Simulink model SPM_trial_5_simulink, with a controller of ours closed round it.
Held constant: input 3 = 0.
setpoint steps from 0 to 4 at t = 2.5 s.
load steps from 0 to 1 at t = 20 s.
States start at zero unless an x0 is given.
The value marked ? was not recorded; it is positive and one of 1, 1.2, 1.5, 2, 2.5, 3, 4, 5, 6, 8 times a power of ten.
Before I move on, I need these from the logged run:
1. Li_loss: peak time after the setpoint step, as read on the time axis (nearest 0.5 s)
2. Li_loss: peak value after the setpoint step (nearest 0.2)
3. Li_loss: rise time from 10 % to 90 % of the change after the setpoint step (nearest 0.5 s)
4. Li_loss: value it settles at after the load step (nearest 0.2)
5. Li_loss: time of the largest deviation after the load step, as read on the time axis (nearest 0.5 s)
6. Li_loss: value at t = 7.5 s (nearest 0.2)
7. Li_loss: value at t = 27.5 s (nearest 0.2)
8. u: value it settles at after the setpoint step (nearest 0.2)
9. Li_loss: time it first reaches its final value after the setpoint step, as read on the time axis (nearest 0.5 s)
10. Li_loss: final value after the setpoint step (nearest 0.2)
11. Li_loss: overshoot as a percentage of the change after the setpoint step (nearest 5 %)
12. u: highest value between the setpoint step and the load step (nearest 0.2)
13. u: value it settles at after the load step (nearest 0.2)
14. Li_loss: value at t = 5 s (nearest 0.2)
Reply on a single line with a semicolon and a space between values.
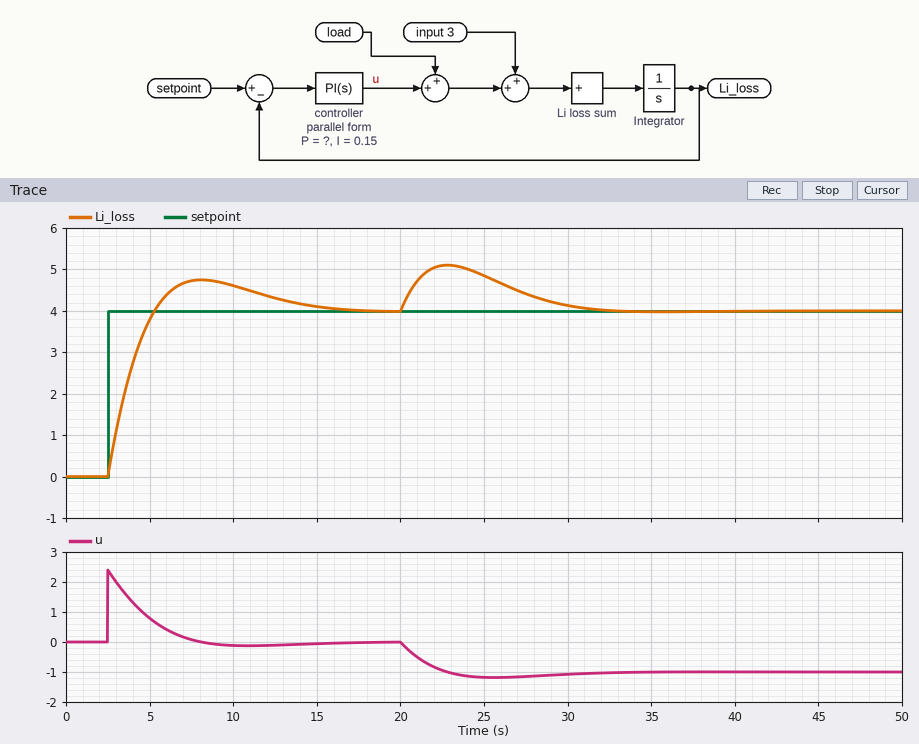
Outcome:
8.0 s; 4.8; 2.0 s; 4.0; 23.0 s; 4.8; 4.4; 0.0; 5.5 s; 4.0; 20 %; 2.4; -1.0; 3.8
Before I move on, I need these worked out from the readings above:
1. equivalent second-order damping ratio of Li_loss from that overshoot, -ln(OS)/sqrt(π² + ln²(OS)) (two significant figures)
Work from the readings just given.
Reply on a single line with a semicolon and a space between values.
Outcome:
0.46
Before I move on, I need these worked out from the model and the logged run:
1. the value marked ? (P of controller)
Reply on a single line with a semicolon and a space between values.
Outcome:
0.6
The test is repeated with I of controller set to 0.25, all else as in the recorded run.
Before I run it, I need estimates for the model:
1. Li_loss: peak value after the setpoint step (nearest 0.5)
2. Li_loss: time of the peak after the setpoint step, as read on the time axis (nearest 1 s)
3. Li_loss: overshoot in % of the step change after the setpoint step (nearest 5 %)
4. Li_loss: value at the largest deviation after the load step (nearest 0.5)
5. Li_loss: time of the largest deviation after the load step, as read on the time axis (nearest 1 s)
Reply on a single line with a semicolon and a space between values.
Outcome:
5.0; 7 s; 25 %; 5.0; 22 s
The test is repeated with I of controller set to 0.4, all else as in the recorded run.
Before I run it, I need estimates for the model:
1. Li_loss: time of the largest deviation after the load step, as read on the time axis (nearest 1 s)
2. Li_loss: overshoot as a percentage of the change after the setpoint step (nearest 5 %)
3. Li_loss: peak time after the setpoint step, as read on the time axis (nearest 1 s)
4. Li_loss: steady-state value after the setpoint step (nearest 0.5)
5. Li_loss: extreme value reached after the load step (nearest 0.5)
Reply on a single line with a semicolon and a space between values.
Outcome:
22 s; 30 %; 6 s; 4.0; 5.0
